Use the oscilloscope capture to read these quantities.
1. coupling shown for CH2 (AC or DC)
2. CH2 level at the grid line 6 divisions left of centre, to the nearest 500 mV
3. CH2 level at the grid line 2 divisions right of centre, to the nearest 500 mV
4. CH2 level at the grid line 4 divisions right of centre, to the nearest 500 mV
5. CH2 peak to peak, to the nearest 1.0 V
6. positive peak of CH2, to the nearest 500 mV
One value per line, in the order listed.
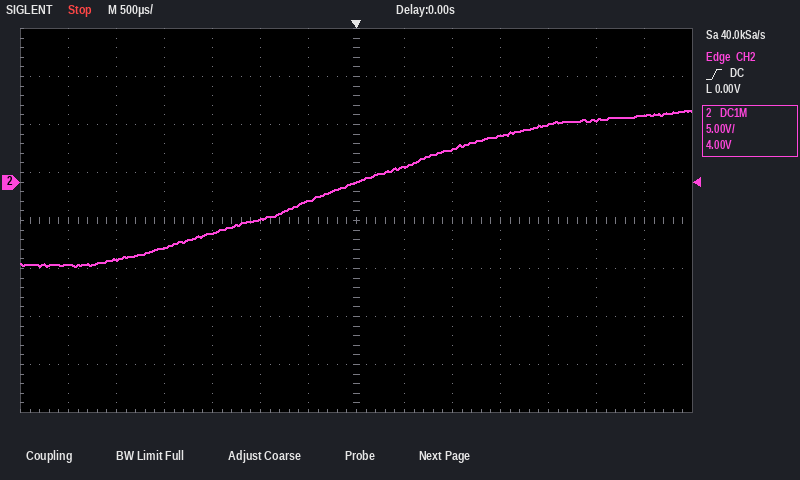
DC
-8.5 V
3.5 V
6.0 V
16.0 V
7.5 V
